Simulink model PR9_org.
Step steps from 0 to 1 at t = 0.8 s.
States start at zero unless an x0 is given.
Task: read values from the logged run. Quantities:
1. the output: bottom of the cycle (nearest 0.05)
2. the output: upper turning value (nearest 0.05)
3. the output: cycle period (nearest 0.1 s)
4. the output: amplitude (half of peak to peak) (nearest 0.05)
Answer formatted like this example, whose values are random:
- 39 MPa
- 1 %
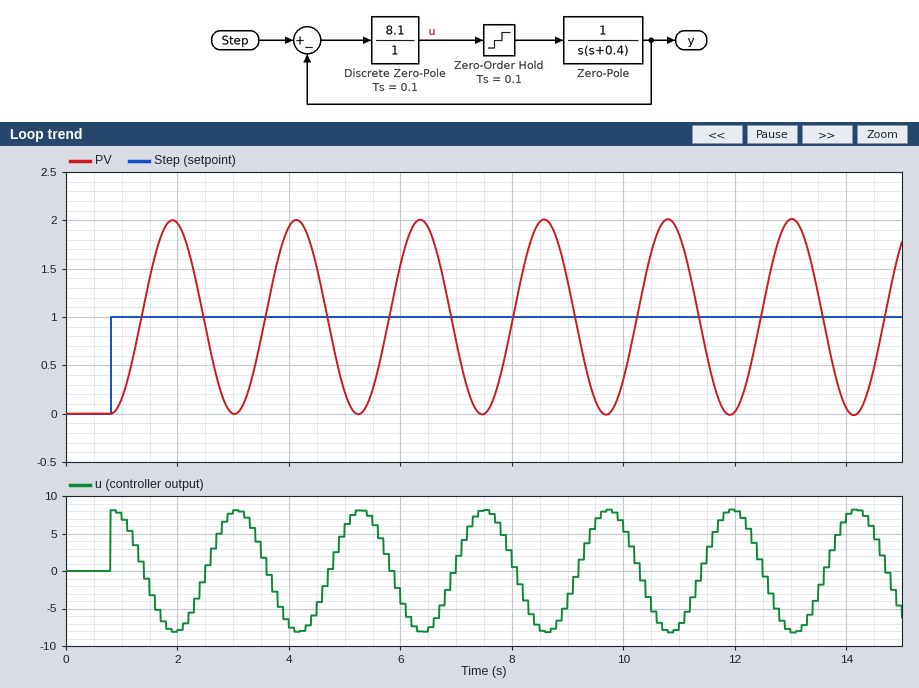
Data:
- 0.00
- 2.00
- 2.2 s
- 1.00
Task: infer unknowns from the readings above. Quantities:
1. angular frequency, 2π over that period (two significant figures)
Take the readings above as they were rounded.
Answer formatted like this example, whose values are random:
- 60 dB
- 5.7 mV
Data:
- 2.9 rad/s
